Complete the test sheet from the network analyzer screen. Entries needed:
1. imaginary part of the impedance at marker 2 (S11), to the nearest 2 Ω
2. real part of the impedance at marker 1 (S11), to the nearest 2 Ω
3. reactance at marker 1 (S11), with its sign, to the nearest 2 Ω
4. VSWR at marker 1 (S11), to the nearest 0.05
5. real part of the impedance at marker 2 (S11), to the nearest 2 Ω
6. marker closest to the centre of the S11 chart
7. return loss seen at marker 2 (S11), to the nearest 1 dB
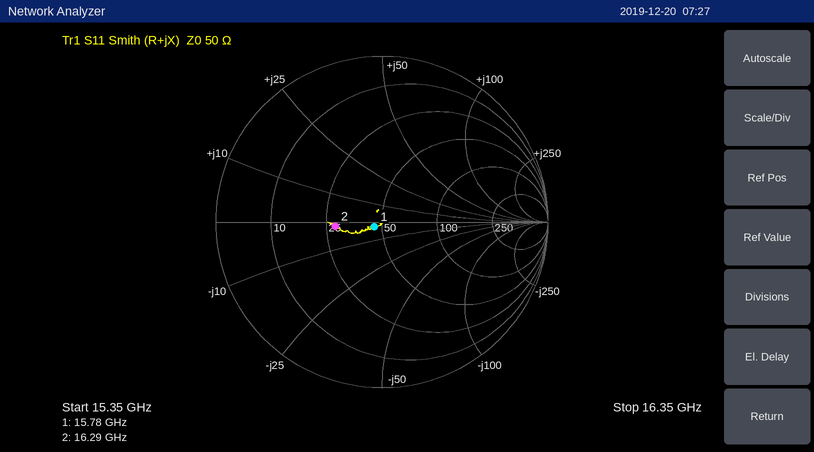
-2 Ω
46 Ω
-2 Ω
1.10
28 Ω
marker 1
11 dB
